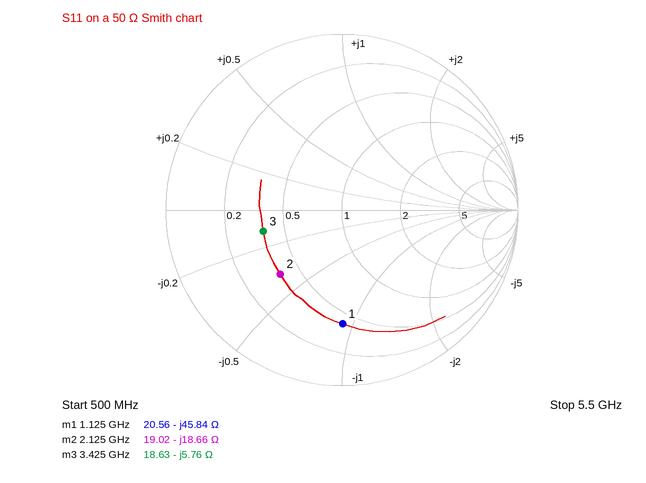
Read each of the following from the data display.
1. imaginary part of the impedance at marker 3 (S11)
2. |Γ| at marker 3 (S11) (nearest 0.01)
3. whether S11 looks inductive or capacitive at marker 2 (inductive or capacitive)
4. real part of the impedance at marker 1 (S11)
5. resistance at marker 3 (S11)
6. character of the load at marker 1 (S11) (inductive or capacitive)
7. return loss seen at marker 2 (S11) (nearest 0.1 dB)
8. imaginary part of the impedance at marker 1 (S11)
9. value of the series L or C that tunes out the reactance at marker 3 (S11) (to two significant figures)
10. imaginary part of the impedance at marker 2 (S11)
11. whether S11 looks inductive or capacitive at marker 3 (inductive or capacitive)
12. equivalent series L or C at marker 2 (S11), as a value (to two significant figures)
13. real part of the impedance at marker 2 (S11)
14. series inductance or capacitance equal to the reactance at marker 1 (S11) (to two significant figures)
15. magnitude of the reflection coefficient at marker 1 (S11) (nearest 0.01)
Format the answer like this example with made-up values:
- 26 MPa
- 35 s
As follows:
- -5.76 Ω
- 0.46
- capacitive
- 20.56 Ω
- 18.63 Ω
- capacitive
- 5.9 dB
- -45.84 Ω
- 270 pH
- -18.66 Ω
- capacitive
- 4.0 pF
- 19.02 Ω
- 3.1 pF
- 0.65
